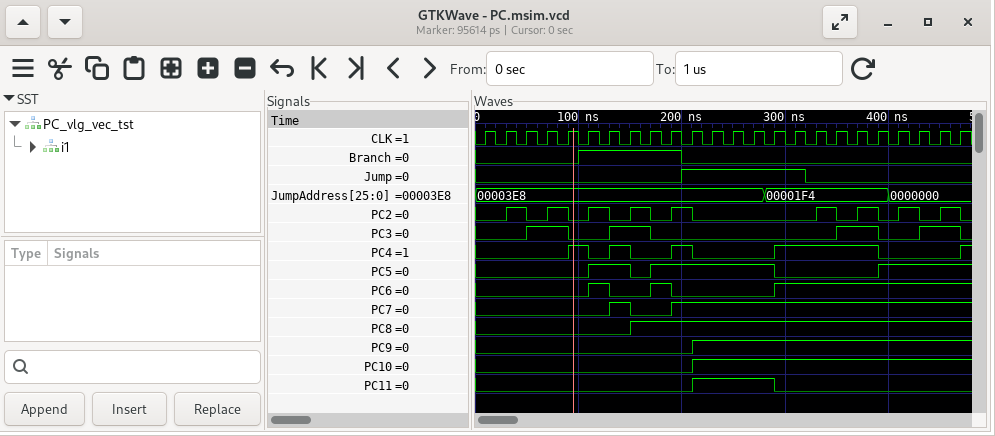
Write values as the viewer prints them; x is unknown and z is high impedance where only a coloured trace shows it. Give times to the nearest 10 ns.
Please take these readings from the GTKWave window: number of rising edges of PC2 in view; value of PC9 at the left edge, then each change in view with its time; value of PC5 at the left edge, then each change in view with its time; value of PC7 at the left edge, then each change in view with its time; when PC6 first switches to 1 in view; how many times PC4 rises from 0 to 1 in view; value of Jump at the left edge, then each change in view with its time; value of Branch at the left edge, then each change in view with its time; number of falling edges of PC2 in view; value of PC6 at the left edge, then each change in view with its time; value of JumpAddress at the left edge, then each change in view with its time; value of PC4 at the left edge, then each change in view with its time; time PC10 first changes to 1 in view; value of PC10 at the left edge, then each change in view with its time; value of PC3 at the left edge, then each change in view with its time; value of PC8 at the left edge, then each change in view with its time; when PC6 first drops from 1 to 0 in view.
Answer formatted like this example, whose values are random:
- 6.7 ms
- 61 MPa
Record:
- 9
- 0, 1 at 210 ns
- 0, 1 at 110 ns, 0 at 150 ns, 1 at 170 ns, 0 at 290 ns, 1 at 390 ns
- 0, 1 at 130 ns, 0 at 150 ns, 1 at 190 ns
- 110 ns
- 5
- 0, 1 at 200 ns, 0 at 320 ns
- 0, 1 at 100 ns, 0 at 200 ns
- 9
- 0, 1 at 110 ns, 0 at 130 ns, 1 at 170 ns, 0 at 190 ns, 1 at 290 ns
- 00003E8, 00001F4 at 280 ns, 0000000 at 400 ns
- 0, 1 at 90 ns, 0 at 110 ns, 1 at 130 ns, 0 at 150 ns, 1 at 190 ns, 0 at 210 ns, 1 at 290 ns, 0 at 390 ns, 1 at 470 ns
- 210 ns
- 0, 1 at 210 ns
- 0, 1 at 50 ns, 0 at 90 ns, 1 at 130 ns, 0 at 170 ns, 1 at 350 ns, 0 at 390 ns, 1 at 430 ns, 0 at 470 ns
- 0, 1 at 150 ns
- 130 ns
